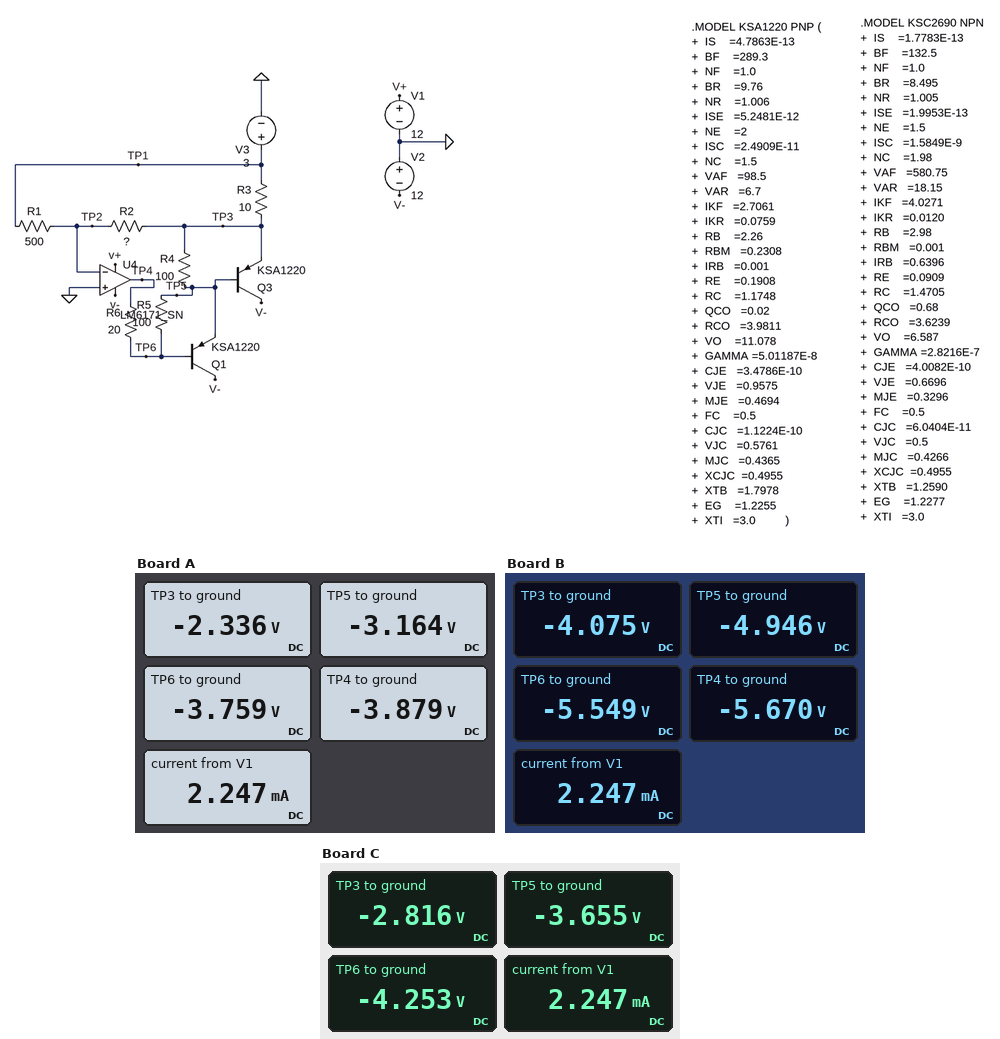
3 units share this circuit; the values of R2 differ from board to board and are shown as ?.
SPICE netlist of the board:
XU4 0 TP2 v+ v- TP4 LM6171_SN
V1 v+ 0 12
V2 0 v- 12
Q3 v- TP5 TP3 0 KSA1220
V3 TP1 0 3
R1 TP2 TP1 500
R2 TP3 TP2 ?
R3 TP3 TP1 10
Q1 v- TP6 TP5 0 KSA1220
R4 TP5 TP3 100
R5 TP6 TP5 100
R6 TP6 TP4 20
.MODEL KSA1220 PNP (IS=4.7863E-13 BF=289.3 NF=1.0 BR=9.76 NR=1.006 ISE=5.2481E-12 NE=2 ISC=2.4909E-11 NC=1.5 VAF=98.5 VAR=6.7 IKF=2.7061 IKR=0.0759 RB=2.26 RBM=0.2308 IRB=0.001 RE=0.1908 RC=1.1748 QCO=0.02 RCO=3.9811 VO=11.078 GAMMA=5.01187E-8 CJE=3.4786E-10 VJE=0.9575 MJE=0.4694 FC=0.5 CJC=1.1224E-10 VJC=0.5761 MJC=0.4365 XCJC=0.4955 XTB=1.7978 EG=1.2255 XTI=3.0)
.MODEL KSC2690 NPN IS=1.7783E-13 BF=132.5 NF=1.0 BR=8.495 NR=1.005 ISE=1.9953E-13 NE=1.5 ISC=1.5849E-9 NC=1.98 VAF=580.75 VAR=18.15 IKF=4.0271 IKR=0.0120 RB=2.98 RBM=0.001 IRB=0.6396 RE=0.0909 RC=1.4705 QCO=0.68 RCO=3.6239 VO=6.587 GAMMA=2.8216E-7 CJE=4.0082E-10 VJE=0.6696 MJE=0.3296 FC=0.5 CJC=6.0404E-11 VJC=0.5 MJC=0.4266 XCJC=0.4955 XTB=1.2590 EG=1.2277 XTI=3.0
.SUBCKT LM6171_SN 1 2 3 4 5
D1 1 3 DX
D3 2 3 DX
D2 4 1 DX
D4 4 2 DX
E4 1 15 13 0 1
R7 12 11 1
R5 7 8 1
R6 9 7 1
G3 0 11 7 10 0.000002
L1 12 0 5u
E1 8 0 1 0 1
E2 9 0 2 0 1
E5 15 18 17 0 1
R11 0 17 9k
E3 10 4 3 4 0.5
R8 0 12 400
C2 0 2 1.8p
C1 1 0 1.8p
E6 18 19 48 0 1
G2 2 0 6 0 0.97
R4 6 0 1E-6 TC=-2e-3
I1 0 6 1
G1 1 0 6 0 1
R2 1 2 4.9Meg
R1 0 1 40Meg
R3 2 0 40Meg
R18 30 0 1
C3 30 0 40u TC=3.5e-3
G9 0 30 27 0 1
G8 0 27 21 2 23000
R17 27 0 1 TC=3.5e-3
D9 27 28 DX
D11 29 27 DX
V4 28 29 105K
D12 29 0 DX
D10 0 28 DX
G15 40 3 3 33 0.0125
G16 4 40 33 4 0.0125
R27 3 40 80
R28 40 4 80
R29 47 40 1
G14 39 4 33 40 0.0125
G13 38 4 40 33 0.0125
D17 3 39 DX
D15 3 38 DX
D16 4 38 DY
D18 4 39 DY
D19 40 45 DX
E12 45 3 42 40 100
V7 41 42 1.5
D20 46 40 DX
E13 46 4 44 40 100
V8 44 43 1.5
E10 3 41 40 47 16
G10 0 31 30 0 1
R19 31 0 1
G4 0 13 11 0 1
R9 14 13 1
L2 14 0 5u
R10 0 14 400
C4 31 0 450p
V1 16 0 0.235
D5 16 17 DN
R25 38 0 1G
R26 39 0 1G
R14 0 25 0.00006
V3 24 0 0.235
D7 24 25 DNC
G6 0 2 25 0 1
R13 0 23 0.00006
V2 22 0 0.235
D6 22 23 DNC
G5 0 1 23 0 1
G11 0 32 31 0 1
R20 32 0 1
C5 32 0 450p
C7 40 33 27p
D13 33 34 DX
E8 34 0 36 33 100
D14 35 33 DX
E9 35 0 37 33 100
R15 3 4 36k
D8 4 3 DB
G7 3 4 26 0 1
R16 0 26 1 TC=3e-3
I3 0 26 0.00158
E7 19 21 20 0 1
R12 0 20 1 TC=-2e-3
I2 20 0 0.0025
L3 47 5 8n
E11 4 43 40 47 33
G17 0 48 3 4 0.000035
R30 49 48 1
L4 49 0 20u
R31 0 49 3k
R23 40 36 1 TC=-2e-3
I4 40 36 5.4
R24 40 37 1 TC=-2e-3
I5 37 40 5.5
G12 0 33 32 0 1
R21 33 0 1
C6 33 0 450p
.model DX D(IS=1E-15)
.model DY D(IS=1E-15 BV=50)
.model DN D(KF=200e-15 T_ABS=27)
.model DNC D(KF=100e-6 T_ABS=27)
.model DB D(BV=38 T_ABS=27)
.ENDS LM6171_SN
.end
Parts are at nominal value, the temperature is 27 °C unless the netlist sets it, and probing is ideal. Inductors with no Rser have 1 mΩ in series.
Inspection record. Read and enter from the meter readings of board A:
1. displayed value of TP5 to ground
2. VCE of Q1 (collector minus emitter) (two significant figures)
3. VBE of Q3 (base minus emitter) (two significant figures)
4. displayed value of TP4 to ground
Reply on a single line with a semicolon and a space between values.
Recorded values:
-3.164 V; -8.8 V; -830 mV; -3.879 V
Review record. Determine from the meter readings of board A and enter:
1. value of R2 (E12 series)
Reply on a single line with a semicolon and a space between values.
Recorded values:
390 Ω
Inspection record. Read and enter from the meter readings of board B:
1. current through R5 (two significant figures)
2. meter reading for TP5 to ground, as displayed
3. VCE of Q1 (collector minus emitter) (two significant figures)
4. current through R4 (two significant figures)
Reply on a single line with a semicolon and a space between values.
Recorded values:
6.0 mA; -4.946 V; -7.1 V; 8.7 mA
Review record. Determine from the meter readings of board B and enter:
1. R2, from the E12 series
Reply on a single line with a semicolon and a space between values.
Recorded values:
680 Ω
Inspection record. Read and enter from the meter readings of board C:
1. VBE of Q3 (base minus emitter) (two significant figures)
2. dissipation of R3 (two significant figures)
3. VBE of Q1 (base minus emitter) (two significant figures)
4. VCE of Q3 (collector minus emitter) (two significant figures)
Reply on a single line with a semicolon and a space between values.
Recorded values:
-840 mV; 3.4 W; -600 mV; -9.2 V
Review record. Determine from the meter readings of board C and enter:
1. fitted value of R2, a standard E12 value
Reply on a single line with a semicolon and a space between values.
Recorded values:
470 Ω
